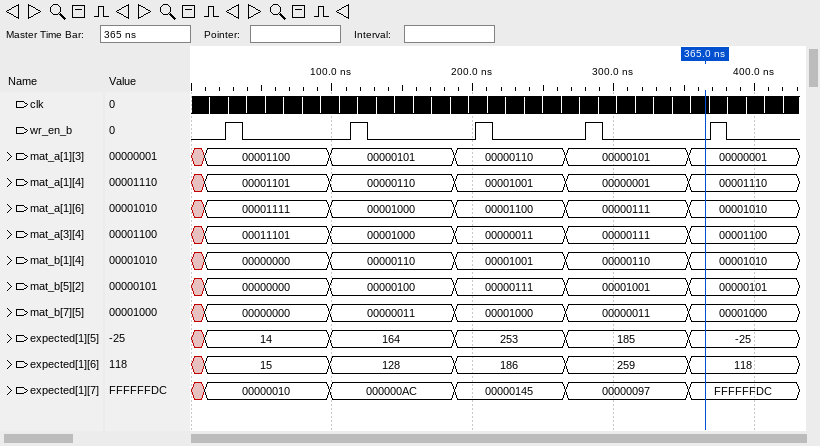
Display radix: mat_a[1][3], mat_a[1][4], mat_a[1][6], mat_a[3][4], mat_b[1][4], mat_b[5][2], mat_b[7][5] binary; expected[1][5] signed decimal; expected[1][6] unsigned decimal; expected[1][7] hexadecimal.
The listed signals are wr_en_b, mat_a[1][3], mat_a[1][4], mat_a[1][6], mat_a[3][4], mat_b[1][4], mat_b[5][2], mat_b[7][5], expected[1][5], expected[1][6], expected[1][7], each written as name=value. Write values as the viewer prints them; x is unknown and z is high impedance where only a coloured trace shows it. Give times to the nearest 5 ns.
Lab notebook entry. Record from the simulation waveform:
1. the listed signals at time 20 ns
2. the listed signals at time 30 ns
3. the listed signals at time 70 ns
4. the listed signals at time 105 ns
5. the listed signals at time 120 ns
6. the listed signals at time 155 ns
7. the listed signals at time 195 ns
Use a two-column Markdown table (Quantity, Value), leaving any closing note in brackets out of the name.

| Quantity | Value |
|---|---|
| the listed signals at time 20 ns | wr_en_b=0, mat_a[1][3]=00001100, mat_a[1][4]=00001101, mat_a[1][6]=00001111, mat_a[3][4]=00011101, mat_b[1][4]=00000000, mat_b[5][2]=00000000, mat_b[7][5]=00000000, expected[1][5]=14, expected[1][6]=15, expected[1][7]=00000010 |
| the listed signals at time 30 ns | wr_en_b=1, mat_a[1][3]=00001100, mat_a[1][4]=00001101, mat_a[1][6]=00001111, mat_a[3][4]=00011101, mat_b[1][4]=00000000, mat_b[5][2]=00000000, mat_b[7][5]=00000000, expected[1][5]=14, expected[1][6]=15, expected[1][7]=00000010 |
| the listed signals at time 70 ns | wr_en_b=0, mat_a[1][3]=00001100, mat_a[1][4]=00001101, mat_a[1][6]=00001111, mat_a[3][4]=00011101, mat_b[1][4]=00000000, mat_b[5][2]=00000000, mat_b[7][5]=00000000, expected[1][5]=14, expected[1][6]=15, expected[1][7]=00000010 |
| the listed signals at time 105 ns | wr_en_b=0, mat_a[1][3]=00000101, mat_a[1][4]=00000110, mat_a[1][6]=00001000, mat_a[3][4]=00001000, mat_b[1][4]=00000110, mat_b[5][2]=00000100, mat_b[7][5]=00000011, expected[1][5]=164, expected[1][6]=128, expected[1][7]=000000AC |
| the listed signals at time 120 ns | wr_en_b=1, mat_a[1][3]=00000101, mat_a[1][4]=00000110, mat_a[1][6]=00001000, mat_a[3][4]=00001000, mat_b[1][4]=00000110, mat_b[5][2]=00000100, mat_b[7][5]=00000011, expected[1][5]=164, expected[1][6]=128, expected[1][7]=000000AC |
| the listed signals at time 155 ns | wr_en_b=0, mat_a[1][3]=00000101, mat_a[1][4]=00000110, mat_a[1][6]=00001000, mat_a[3][4]=00001000, mat_b[1][4]=00000110, mat_b[5][2]=00000100, mat_b[7][5]=00000011, expected[1][5]=164, expected[1][6]=128, expected[1][7]=000000AC |
| the listed signals at time 195 ns | wr_en_b=0, mat_a[1][3]=00000110, mat_a[1][4]=00001001, mat_a[1][6]=00001100, mat_a[3][4]=00000011, mat_b[1][4]=00001001, mat_b[5][2]=00000111, mat_b[7][5]=00001000, expected[1][5]=253, expected[1][6]=186, expected[1][7]=00000145 |
